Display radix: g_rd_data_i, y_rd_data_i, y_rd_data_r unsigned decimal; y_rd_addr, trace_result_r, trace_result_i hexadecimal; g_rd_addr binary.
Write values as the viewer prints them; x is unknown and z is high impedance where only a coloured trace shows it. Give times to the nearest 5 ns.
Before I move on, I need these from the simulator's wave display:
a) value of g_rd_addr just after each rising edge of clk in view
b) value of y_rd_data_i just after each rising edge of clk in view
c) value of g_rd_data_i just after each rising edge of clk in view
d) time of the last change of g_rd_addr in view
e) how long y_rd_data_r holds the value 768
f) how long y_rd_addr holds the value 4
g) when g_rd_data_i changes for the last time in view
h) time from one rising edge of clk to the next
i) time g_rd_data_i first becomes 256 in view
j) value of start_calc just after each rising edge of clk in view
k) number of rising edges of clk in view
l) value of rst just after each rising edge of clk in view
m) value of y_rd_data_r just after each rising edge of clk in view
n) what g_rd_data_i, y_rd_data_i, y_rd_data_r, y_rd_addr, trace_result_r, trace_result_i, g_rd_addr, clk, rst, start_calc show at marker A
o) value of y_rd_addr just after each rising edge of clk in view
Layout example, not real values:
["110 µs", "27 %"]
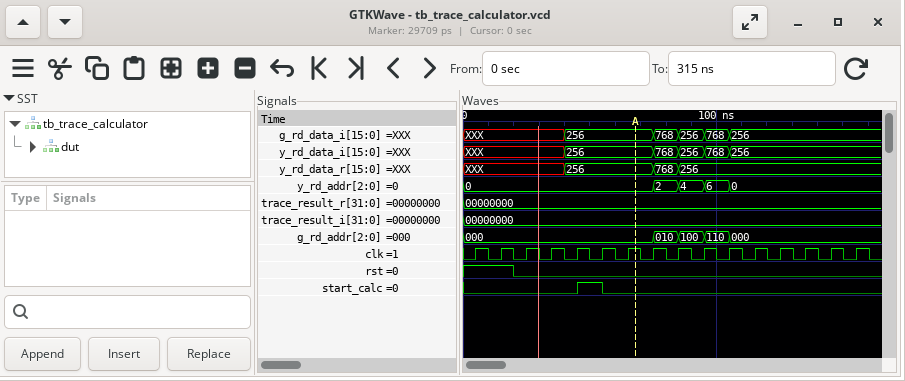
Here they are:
["000, 000, 000, 000, 000, 000, 000, 010, 100, 110, 000, 000, 000, 000, 000, 000", "XXX, XXX, XXX, XXX, 256, 256, 256, 768, 256, 768, 256, 256, 256, 256, 256, 256", "XXX, XXX, XXX, XXX, 256, 256, 256, 768, 256, 768, 256, 256, 256, 256, 256, 256", "105 ns", "10 ns", "10 ns", "105 ns", "10 ns", "40 ns", "0 0 0 0 1 0 0 0 0 0 0 0 0 0 0 0", "16", "1 1 0 0 0 0 0 0 0 0 0 0 0 0 0 0", "XXX, XXX, XXX, XXX, 256, 256, 256, 768, 256, 256, 256, 256, 256, 256, 256, 256", "g_rd_data_i=256, y_rd_data_i=256, y_rd_data_r=256, y_rd_addr=0, trace_result_r=00000000, trace_result_i=00000000, g_rd_addr=000, clk=1, rst=0, start_calc=0", "0, 0, 0, 0, 0, 0, 0, 2, 4, 6, 0, 0, 0, 0, 0, 0"]
